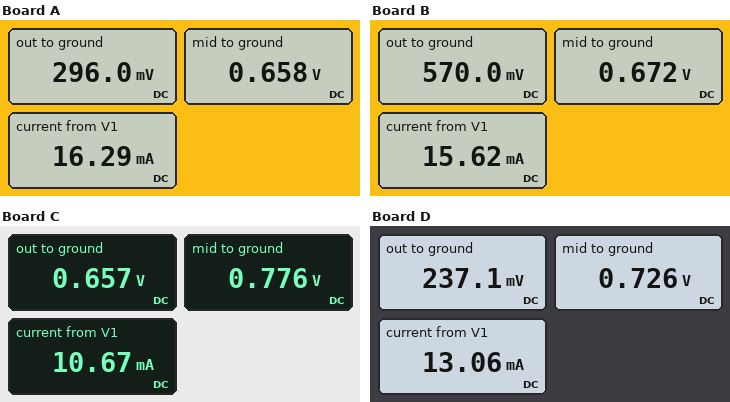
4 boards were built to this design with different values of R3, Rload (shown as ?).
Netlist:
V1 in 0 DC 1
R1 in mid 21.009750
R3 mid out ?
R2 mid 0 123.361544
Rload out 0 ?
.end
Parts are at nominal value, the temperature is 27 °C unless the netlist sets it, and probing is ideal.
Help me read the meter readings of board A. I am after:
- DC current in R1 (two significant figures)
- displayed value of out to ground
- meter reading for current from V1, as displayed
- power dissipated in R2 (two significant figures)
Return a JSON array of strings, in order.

["16 mA", "296.0 mV", "16.29 mA", "3.5 mW"]
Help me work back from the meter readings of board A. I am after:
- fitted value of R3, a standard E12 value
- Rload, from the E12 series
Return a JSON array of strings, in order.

["33 Ω", "27 Ω"]
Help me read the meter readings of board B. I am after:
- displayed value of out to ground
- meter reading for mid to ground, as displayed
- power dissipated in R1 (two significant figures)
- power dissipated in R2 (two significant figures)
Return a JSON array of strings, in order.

["570.0 mV", "0.672 V", "5.1 mW", "3.7 mW"]
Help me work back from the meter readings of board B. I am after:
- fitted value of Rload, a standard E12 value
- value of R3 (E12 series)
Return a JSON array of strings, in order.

["56 Ω", "10 Ω"]
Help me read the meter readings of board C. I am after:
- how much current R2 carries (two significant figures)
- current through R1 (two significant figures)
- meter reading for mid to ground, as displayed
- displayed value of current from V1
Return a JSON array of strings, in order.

["6.3 mA", "11 mA", "0.776 V", "10.67 mA"]
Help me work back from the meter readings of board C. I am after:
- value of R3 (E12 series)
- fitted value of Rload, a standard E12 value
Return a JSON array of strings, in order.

["27 Ω", "150 Ω"]
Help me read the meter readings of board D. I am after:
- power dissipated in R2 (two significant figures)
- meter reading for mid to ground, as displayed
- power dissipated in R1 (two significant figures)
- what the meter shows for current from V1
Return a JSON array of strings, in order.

["4.3 mW", "0.726 V", "3.6 mW", "13.06 mA"]
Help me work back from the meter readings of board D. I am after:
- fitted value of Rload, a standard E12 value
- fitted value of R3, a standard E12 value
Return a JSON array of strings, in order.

["33 Ω", "68 Ω"]
